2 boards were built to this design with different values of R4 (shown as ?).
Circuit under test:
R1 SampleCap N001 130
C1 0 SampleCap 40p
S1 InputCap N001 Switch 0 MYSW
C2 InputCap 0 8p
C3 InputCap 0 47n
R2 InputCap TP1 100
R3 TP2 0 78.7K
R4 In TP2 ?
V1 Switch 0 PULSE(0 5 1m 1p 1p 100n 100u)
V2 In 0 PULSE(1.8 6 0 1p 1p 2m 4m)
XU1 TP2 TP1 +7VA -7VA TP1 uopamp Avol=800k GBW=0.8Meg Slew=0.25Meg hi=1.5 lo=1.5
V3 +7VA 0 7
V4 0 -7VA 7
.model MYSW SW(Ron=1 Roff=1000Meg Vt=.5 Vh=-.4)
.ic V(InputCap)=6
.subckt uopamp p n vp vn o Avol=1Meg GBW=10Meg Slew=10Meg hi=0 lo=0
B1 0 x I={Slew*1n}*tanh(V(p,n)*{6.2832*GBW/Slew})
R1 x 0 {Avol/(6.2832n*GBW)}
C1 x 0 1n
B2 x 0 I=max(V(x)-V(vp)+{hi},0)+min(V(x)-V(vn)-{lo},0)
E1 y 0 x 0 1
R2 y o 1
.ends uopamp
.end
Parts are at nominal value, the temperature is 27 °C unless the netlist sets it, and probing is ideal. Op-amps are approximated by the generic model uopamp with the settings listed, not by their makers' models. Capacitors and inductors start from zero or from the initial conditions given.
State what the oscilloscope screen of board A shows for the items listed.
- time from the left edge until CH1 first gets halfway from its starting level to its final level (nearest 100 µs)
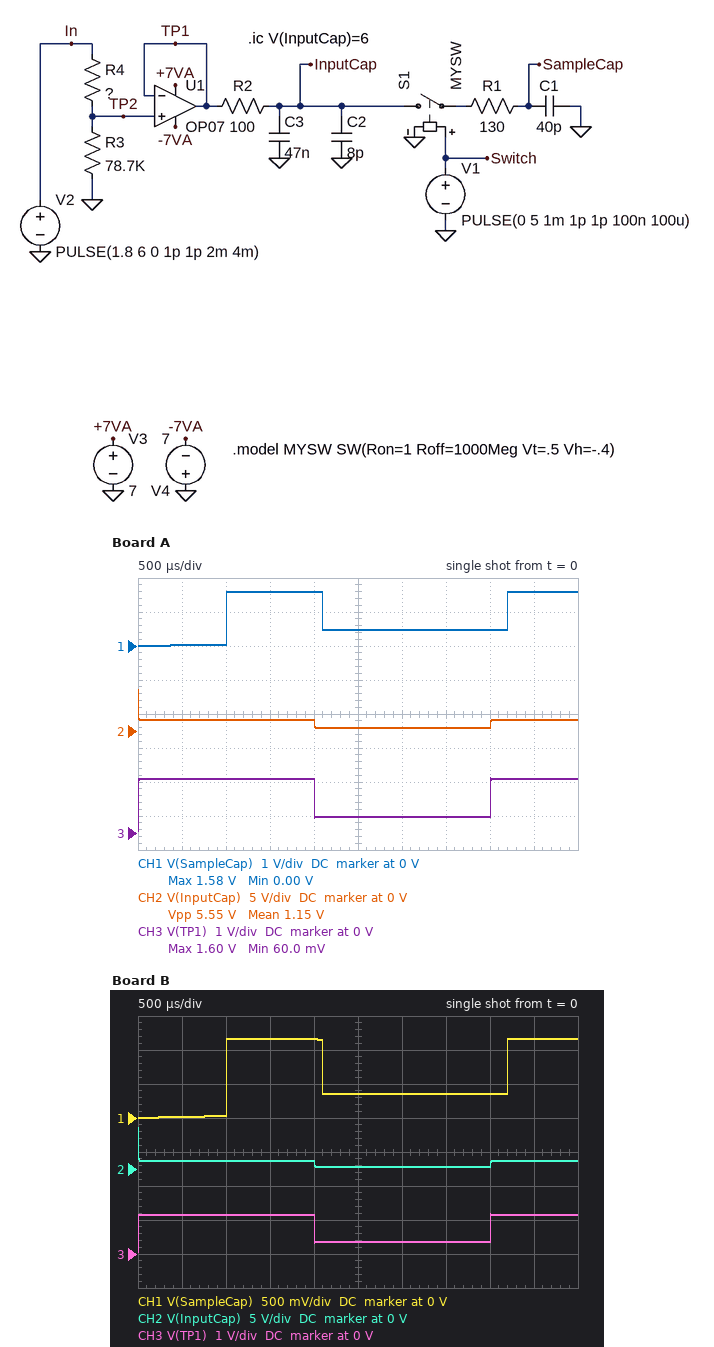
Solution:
1.0 ms
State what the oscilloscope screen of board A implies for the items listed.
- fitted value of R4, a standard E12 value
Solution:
220 kΩ
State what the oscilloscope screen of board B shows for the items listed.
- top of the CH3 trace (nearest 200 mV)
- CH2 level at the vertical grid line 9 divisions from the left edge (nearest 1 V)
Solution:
1.2 V
1 V
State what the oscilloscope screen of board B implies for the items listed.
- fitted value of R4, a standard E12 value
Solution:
330 kΩ
